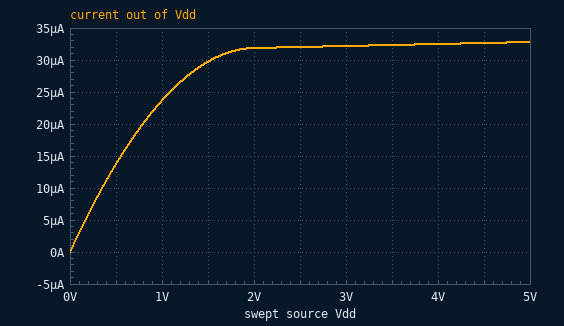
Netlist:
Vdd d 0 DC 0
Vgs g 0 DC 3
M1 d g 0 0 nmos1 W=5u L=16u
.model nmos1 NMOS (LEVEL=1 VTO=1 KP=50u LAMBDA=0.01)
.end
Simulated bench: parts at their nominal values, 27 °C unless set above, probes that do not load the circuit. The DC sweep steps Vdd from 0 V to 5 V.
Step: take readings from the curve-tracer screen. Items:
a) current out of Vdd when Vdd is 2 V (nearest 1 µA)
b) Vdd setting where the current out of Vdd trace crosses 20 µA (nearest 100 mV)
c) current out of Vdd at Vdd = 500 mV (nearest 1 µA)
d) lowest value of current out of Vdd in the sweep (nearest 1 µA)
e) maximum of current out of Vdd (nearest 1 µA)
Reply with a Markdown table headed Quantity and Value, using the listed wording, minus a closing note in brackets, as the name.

| Quantity | Value |
|---|---|
| current out of Vdd when Vdd is 2 V | 32 µA |
| Vdd setting where the current out of Vdd trace crosses 20 µA | 800 mV |
| current out of Vdd at Vdd = 500 mV | 14 µA |
| lowest value of current out of Vdd in the sweep | 0 A |
| maximum of current out of Vdd | 33 µA |
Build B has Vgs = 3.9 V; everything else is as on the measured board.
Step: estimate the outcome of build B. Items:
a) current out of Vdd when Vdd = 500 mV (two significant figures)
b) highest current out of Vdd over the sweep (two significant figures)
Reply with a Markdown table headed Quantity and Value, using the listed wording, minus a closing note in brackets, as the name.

| Quantity | Value |
|---|---|
| current out of Vdd when Vdd = 500 mV | 21 µA |
| highest current out of Vdd over the sweep | 69 µA |
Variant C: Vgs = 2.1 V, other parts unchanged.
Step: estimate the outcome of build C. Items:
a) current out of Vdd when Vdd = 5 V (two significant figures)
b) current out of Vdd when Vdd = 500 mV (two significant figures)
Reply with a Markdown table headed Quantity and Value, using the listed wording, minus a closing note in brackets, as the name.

| Quantity | Value |
|---|---|
| current out of Vdd when Vdd = 5 V | 9.9 µA |
| current out of Vdd when Vdd = 500 mV | 6.7 µA |
